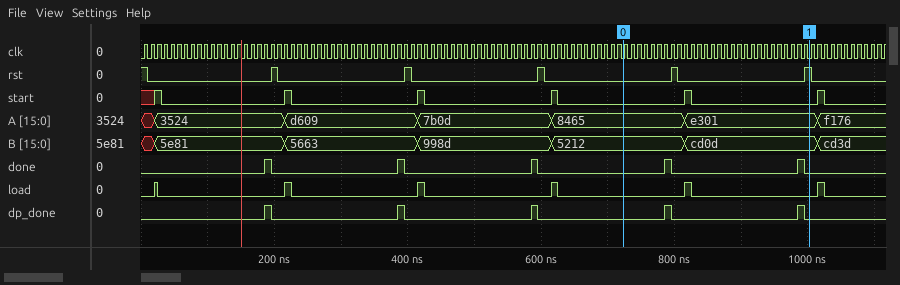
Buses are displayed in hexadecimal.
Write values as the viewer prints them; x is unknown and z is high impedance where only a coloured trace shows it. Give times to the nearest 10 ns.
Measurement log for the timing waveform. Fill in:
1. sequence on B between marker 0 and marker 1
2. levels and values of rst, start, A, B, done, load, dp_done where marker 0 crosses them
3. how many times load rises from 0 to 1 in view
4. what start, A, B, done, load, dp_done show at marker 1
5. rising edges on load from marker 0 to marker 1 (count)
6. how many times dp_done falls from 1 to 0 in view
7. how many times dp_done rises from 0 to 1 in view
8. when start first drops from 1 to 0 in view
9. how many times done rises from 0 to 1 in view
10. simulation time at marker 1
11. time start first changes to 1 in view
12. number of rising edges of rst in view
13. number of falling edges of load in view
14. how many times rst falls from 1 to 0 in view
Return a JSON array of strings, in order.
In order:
["5212, cd0d", "rst=0, start=0, A=8465, B=5212, done=0, load=0, dp_done=0", "6", "start=0, A=e301, B=cd0d, done=0, load=0, dp_done=0", "1", "5", "5", "30 ns", "5", "1000 ns", "20 ns", "5", "6", "6"]
